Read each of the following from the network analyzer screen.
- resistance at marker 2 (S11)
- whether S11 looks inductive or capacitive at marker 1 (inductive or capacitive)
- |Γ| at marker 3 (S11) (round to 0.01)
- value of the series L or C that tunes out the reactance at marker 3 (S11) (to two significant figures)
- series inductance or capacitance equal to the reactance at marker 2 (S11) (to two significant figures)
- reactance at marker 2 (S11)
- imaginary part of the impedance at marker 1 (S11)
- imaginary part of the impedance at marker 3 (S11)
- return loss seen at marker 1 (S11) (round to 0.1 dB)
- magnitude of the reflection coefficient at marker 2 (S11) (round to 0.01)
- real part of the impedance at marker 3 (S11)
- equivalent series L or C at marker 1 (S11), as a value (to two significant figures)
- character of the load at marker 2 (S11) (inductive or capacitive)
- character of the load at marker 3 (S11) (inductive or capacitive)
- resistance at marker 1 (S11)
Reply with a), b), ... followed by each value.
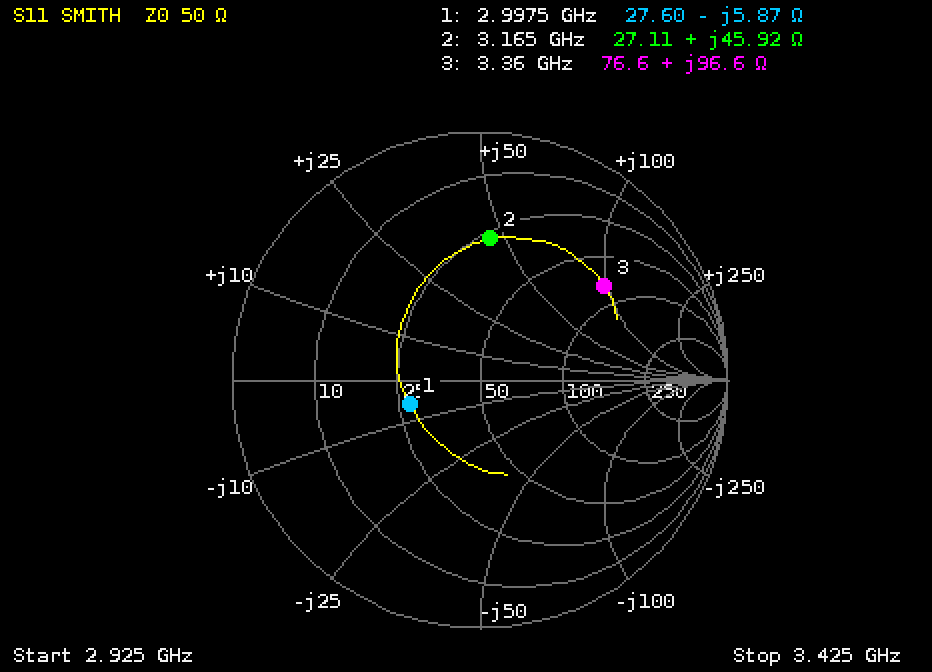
a) 27.11 Ω
b) capacitive
c) 0.63
d) 490 fF
e) 2.3 nH
f) +45.92 Ω
g) -5.87 Ω
h) +96.6 Ω
i) 10.5 dB
j) 0.57
k) 76.6 Ω
l) 9.0 pF
m) inductive
n) inductive
o) 27.60 Ω
